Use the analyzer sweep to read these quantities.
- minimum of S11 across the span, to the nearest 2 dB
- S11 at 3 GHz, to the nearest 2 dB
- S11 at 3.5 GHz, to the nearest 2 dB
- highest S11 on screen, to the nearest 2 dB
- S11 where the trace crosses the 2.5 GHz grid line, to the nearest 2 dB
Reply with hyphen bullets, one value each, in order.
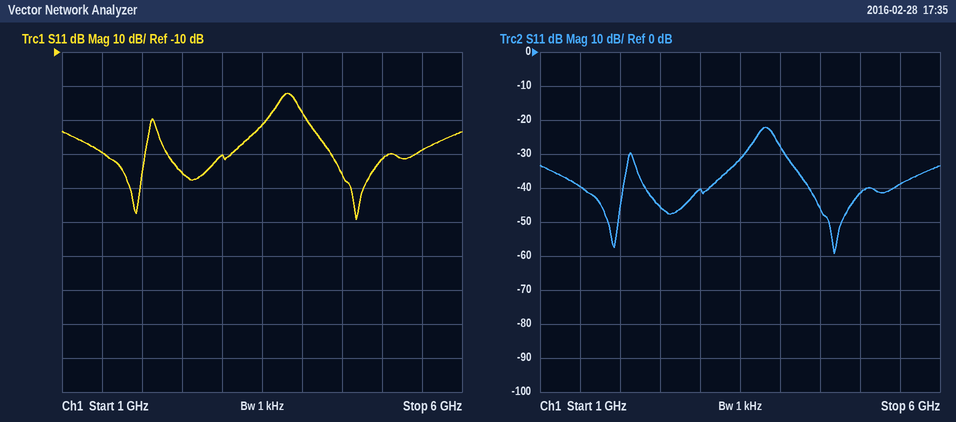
- -60 dB
- -40 dB
- -32 dB
- -22 dB
- -46 dB
